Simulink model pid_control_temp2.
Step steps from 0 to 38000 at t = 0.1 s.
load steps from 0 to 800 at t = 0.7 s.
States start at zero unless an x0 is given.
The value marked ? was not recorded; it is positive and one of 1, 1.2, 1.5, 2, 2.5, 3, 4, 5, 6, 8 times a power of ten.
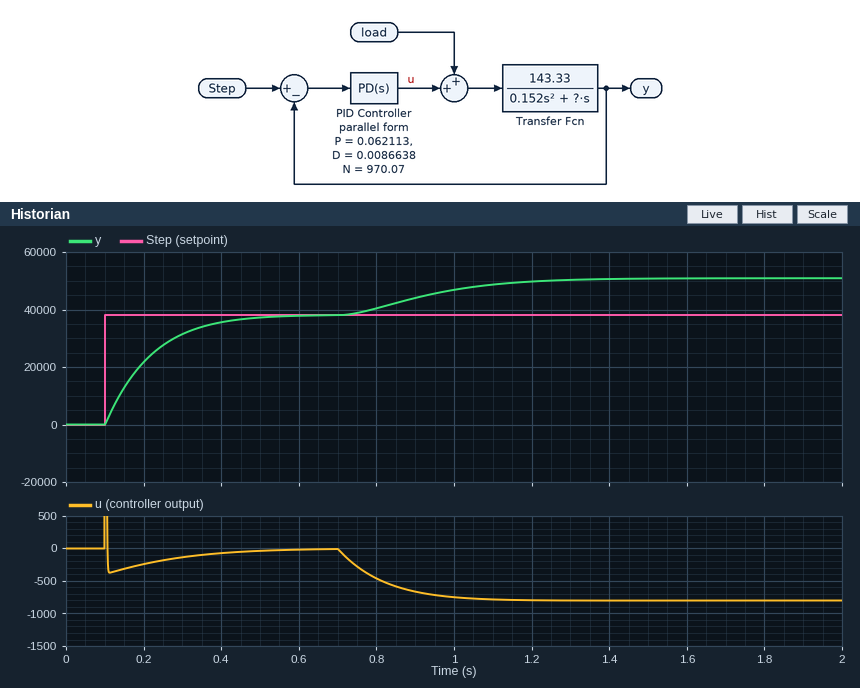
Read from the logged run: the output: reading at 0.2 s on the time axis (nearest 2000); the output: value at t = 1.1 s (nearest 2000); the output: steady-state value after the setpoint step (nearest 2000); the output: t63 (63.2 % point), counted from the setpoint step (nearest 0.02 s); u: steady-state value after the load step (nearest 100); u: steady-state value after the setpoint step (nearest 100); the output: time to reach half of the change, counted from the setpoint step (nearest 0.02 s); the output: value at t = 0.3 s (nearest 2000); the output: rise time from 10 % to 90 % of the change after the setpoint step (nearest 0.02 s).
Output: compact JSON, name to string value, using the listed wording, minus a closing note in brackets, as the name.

{"the output: reading at 0.2 s on the time axis": "22000", "the output: value at t = 1.1 s": "48000", "the output: steady-state value after the setpoint step": "38000", "the output: t63 (63.2 % point), counted from the setpoint step": "0.12 s", "u: steady-state value after the load step": "-800", "u: steady-state value after the setpoint step": "0", "the output: time to reach half of the change, counted from the setpoint step": "0.08 s", "the output: value at t = 0.3 s": "32000", "the output: rise time from 10 % to 90 % of the change after the setpoint step": "0.24 s"}
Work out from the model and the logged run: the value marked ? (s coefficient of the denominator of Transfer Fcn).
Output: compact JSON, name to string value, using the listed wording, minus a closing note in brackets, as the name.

{"the value marked ?": "1"}
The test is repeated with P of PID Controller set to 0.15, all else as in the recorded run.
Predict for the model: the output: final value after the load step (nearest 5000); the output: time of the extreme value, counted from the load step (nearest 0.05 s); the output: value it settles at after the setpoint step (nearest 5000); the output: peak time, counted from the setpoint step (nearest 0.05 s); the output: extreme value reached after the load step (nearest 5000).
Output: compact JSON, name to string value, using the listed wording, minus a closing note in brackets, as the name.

{"the output: final value after the load step": "45000", "the output: time of the extreme value, counted from the load step": "0.35 s", "the output: value it settles at after the setpoint step": "40000", "the output: peak time, counted from the setpoint step": "0.25 s", "the output: extreme value reached after the load step": "45000"}
